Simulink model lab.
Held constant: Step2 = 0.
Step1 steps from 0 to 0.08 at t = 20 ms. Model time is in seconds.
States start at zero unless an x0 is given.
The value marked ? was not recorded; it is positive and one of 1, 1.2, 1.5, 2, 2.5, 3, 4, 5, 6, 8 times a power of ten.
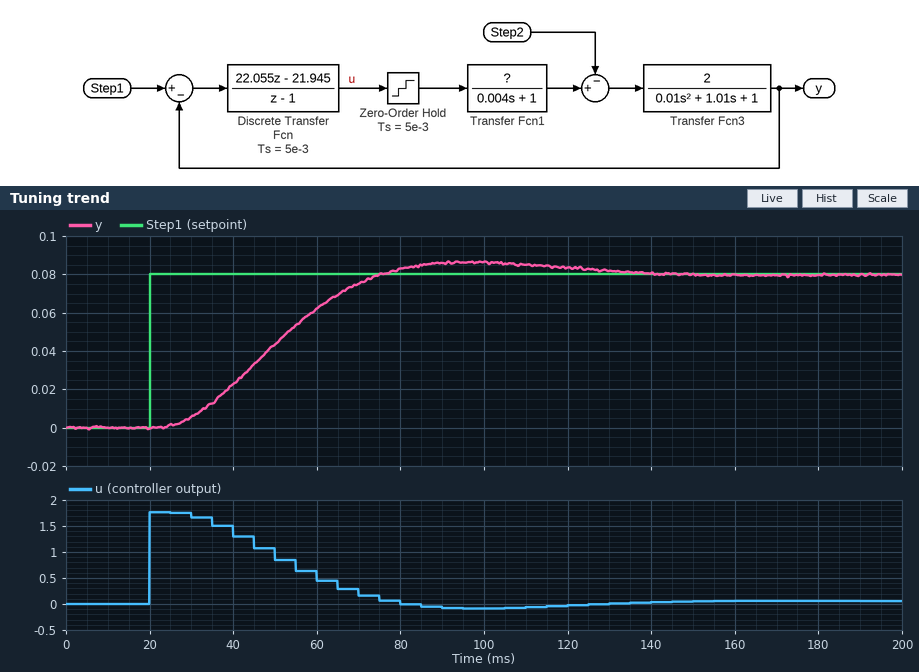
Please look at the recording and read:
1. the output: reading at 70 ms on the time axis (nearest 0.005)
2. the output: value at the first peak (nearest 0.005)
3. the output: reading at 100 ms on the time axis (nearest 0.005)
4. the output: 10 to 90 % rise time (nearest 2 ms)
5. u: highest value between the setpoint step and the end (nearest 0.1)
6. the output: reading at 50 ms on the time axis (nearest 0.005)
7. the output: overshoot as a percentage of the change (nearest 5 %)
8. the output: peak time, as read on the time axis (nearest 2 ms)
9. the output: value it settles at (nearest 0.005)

0.075
0.085
0.085
36 ms
1.8
0.045
10 %
96 ms
0.080
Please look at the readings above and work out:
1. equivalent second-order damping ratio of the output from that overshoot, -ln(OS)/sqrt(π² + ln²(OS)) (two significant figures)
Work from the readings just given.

0.59
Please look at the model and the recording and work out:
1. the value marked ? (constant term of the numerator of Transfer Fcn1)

0.8
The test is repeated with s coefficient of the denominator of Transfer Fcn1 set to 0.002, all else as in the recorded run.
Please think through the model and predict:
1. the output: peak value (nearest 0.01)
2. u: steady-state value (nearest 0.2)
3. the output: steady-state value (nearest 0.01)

0.08
0.0
0.08
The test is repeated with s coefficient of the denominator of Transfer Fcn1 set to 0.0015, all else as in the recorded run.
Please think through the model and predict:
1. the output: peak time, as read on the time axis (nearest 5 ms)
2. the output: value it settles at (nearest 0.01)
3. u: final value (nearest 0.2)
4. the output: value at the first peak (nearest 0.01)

100 ms
0.08
0.0
0.08
